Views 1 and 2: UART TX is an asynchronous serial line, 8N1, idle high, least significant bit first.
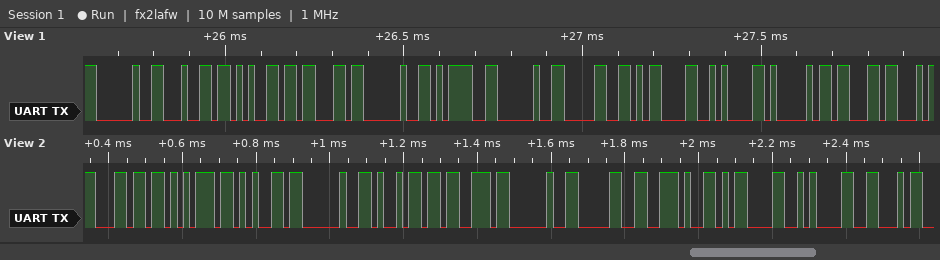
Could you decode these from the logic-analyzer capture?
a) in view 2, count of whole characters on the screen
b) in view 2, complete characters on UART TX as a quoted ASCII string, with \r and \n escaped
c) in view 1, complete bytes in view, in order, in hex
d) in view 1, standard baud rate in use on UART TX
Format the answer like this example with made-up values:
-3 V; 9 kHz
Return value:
12; "lue is 0.\r\nF"; 20 64 65 63 20 3D 20 30 0D 0A 41 63; 57600 baud
